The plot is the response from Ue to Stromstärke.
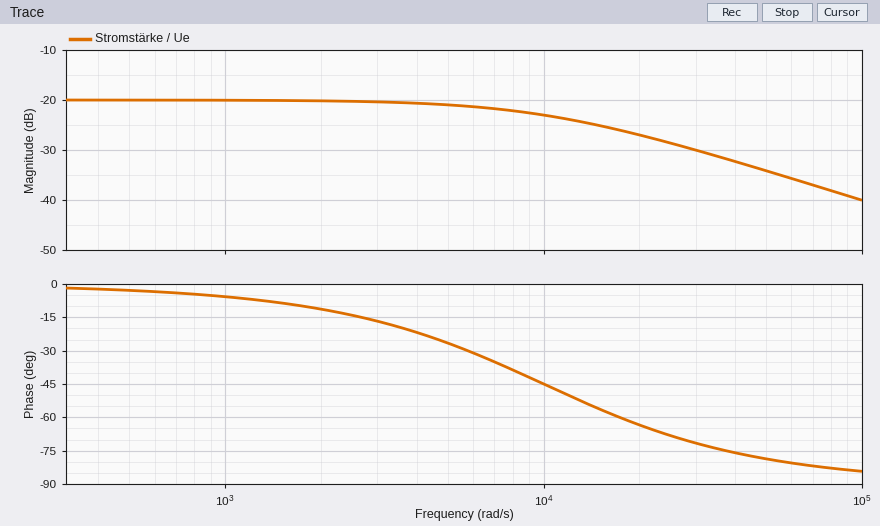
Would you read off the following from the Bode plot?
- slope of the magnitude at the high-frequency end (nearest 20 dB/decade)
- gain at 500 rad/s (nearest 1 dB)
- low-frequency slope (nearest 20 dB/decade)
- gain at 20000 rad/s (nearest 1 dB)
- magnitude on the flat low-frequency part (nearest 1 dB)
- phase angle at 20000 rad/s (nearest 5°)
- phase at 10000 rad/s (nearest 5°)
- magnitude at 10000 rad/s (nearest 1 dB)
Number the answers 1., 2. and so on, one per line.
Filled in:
1. -20 dB/decade
2. -20 dB
3. 0 dB/decade
4. -27 dB
5. -20 dB
6. -65°
7. -45°
8. -23 dB
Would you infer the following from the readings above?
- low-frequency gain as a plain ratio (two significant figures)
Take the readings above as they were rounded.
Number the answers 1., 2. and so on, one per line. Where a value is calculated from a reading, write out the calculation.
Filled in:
1. 10^(-20 / 20) = 0.10
